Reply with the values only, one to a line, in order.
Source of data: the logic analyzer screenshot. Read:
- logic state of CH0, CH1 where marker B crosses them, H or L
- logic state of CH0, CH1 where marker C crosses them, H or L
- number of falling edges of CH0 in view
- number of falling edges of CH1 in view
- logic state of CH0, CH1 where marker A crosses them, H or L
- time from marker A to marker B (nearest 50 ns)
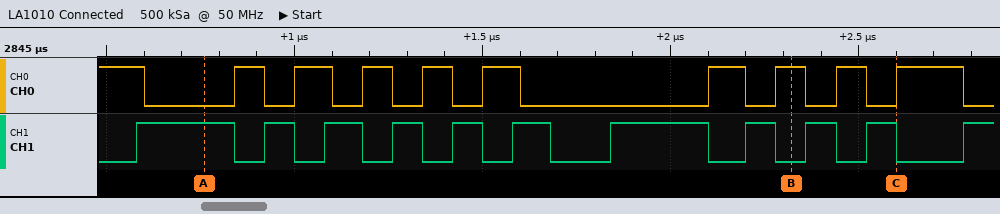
CH0=H, CH1=L
CH0=H, CH1=L
10
10
CH0=L, CH1=H
1550 ns
